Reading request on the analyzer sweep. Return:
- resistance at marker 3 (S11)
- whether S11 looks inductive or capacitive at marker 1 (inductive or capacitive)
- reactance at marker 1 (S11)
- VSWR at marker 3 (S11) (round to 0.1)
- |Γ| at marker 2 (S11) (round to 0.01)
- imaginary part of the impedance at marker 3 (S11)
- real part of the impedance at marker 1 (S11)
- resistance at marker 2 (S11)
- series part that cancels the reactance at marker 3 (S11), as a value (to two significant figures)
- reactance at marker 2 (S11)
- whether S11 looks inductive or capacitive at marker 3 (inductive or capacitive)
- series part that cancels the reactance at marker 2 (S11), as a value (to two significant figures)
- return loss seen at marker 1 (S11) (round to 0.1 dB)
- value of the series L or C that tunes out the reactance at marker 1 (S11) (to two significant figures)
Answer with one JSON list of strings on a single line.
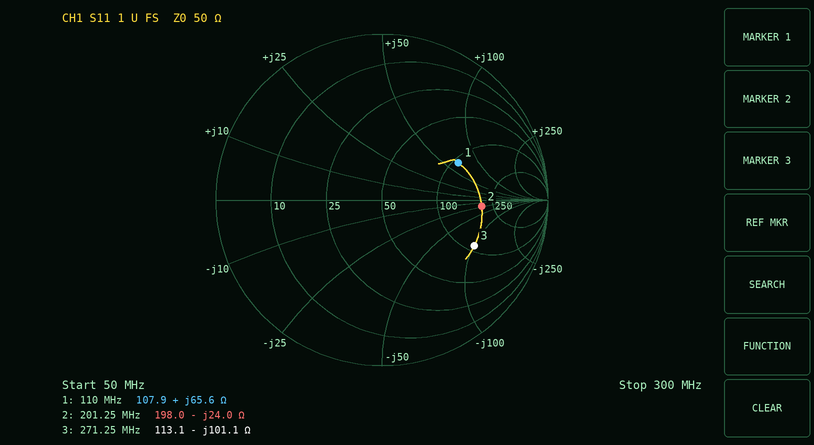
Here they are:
["113.1 Ω", "inductive", "+65.6 Ω", "4.3", "0.60", "-101.1 Ω", "107.9 Ω", "198.0 Ω", "59 nH", "-24.0 Ω", "capacitive", "19 nH", "5.8 dB", "22 pF"]
